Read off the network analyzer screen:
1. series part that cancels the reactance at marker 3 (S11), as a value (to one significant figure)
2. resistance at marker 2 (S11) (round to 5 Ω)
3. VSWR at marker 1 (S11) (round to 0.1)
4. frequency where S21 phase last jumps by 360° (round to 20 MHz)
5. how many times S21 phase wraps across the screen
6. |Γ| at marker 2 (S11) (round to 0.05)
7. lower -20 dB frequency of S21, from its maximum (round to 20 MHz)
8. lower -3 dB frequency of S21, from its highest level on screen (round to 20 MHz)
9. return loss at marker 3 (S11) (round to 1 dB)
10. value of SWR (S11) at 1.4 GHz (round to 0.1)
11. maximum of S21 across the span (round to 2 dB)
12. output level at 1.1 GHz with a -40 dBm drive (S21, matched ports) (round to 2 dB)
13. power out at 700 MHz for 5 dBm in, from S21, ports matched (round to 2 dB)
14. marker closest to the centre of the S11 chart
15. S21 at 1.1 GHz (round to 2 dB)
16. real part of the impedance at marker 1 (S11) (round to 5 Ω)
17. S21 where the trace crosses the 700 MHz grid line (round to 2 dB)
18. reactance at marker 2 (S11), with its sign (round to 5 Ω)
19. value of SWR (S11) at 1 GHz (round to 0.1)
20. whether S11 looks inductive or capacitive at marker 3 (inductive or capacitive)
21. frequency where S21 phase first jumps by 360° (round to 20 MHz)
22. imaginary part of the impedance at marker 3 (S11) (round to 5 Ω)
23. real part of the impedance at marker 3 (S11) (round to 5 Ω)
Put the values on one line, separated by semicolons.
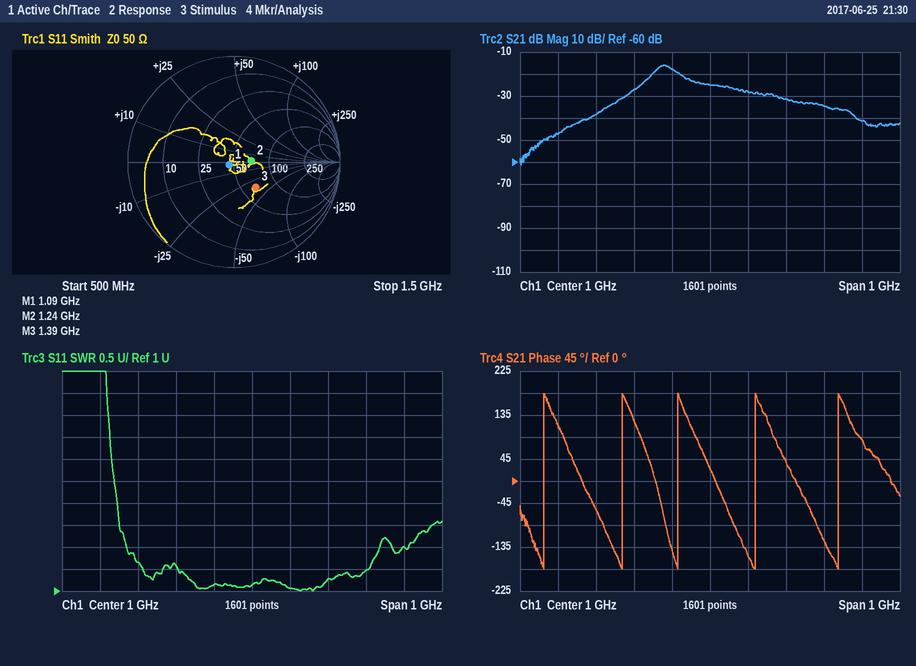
4 nH; 70 Ω; 1.1; 1.34 GHz; 5; 0.15; 720 MHz; 860 MHz; 10 dB; 2.0; -16 dB; -68 dBm; -34 dBm; marker 1; -28 dB; 45 Ω; -38 dB; 0 Ω; 1.1; capacitive; 560 MHz; -35 Ω; 65 Ω
